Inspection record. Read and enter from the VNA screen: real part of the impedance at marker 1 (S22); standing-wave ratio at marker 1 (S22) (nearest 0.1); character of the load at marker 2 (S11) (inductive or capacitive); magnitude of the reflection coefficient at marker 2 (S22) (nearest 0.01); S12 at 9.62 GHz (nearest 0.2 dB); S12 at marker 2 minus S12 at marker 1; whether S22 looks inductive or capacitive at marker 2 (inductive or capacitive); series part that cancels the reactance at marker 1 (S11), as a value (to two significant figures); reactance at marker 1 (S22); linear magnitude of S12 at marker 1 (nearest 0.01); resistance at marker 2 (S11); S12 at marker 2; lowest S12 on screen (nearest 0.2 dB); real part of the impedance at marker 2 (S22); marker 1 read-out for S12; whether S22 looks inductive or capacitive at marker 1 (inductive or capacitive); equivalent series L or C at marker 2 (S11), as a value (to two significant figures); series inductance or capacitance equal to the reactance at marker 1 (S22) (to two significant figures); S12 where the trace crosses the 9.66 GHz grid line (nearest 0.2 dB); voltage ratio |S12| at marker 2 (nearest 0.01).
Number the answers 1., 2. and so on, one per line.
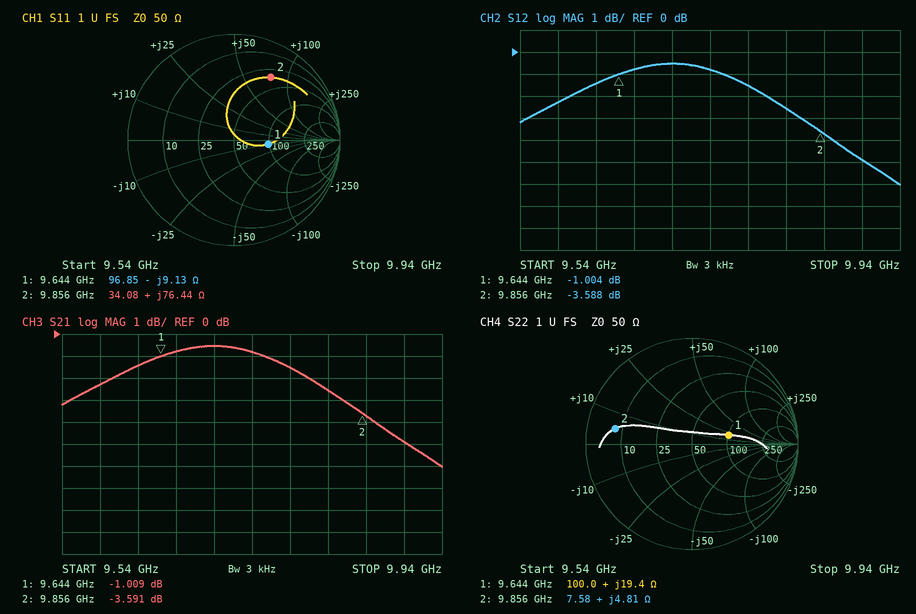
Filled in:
1. 100.0 Ω
2. 2.1
3. inductive
4. 0.74
5. -1.4 dB
6. -2.584 dB
7. inductive
8. 150 pH
9. +19.4 Ω
10. 0.89
11. 34.08 Ω
12. -3.588 dB
13. -6.0 dB
14. 7.58 Ω
15. -1.004 dB
16. inductive
17. 1.2 nH
18. 320 pH
19. -0.8 dB
20. 0.66
